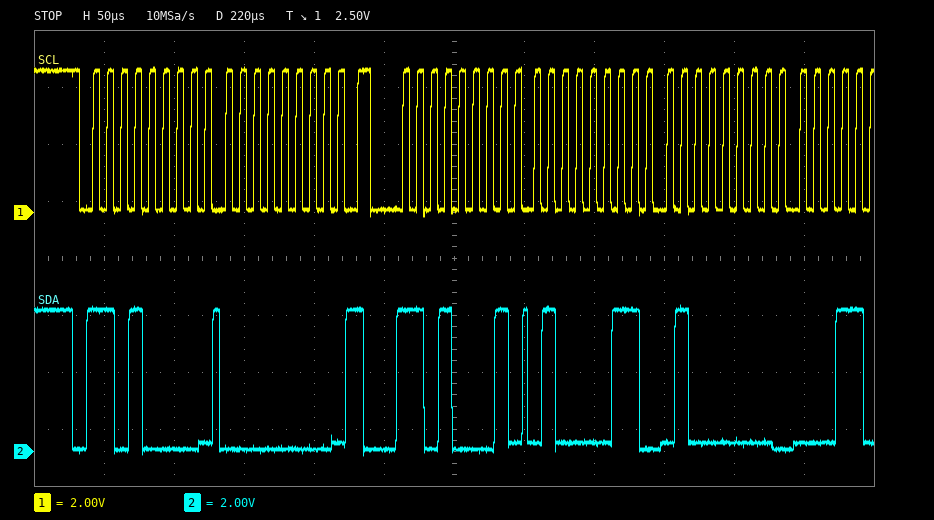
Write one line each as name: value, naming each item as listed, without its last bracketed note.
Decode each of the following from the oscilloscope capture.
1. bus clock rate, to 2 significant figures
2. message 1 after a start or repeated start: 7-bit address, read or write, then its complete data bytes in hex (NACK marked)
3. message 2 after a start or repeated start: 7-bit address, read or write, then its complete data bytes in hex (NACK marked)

bus clock rate, to 2 significant figures: 100 kHz
message 1 after a start or repeated start: 7-bit address, read or write, then its complete data bytes in hex: 0x68 write: 00
message 2 after a start or repeated start: 7-bit address, read or write, then its complete data bytes in hex: 0x68 read: 43 40
